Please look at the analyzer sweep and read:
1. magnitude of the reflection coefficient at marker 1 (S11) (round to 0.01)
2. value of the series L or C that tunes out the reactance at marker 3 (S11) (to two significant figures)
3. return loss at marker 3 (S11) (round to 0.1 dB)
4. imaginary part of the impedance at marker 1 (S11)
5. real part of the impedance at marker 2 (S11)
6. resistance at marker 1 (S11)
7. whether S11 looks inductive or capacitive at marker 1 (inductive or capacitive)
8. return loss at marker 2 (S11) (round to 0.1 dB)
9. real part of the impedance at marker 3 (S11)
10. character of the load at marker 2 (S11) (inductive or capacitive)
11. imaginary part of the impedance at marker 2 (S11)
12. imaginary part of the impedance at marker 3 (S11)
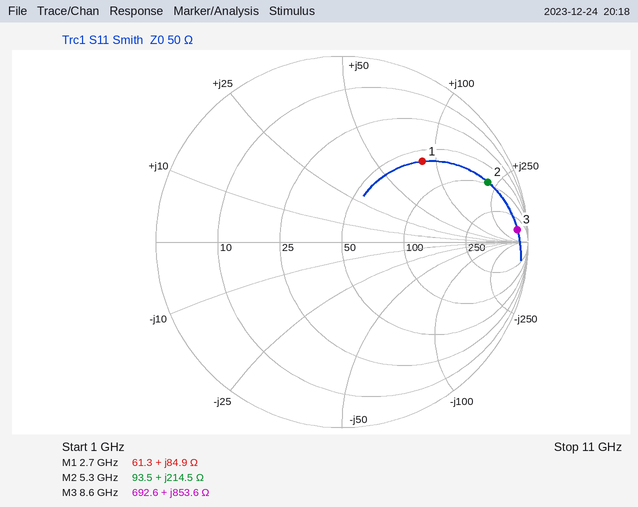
0.61
22 fF
0.5 dB
+84.9 Ω
93.5 Ω
61.3 Ω
inductive
1.4 dB
692.6 Ω
inductive
+214.5 Ω
+853.6 Ω
